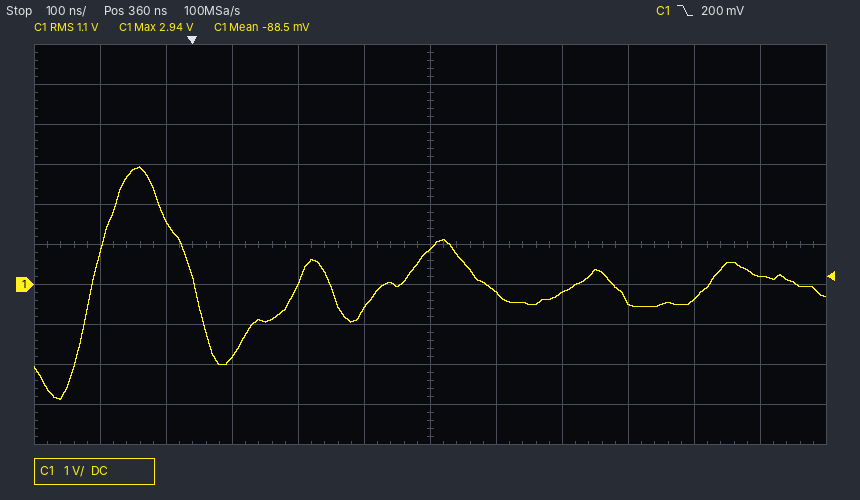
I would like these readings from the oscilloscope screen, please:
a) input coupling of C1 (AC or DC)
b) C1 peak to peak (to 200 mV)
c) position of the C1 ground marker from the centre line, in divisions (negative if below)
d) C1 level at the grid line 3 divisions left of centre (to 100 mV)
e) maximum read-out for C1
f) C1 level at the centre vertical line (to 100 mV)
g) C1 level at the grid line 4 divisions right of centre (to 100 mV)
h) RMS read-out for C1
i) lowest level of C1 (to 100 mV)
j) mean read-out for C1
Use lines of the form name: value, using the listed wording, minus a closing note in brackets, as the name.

input coupling of C1: DC
C1 peak to peak: 5.8 V
position of the C1 ground marker from the centre line, in divisions: -1.0 div
C1 level at the grid line 3 divisions left of centre: -1.8 V
maximum read-out for C1: 2.94 V
C1 level at the centre vertical line: 900 mV
C1 level at the grid line 4 divisions right of centre: -400 mV
RMS read-out for C1: 1.1 V
lowest level of C1: -2.9 V
mean read-out for C1: -88.5 mV
